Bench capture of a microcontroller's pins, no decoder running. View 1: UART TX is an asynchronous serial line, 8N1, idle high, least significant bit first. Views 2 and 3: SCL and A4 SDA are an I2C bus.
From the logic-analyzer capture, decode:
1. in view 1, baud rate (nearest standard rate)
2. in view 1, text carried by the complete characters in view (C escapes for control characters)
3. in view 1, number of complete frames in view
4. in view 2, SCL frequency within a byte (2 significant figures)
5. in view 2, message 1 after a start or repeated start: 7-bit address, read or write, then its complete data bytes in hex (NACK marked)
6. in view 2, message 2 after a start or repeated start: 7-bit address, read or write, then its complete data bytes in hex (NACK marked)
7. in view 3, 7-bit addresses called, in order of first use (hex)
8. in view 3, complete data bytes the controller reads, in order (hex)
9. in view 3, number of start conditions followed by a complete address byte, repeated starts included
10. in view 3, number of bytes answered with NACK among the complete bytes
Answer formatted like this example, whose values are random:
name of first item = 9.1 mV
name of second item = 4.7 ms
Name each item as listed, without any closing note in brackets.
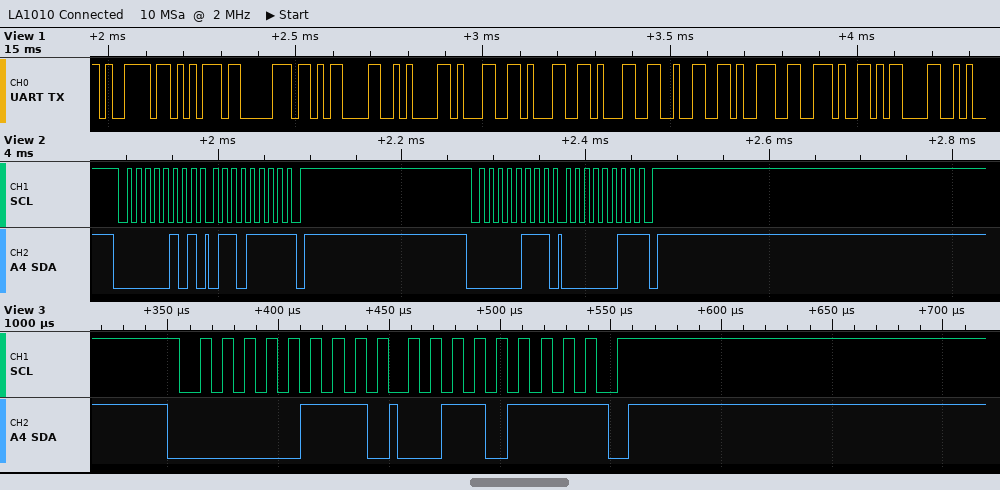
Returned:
in view 1, baud rate = 57600 baud
in view 1, text carried by the complete characters in view = "yup\r\n11129.\r"
in view 1, number of complete frames in view = 12
in view 2, SCL frequency within a byte = 100 kHz
in view 2, message 1 after a start or repeated start: 7-bit address, read or write, then its complete data bytes in hex = 0x02 read: 6F NACK
in view 2, message 2 after a start or repeated start: 7-bit address, read or write, then its complete data bytes in hex = 0x03 read: 03 NACK
in view 3, 7-bit addresses called, in order of first use = 0x03
in view 3, complete data bytes the controller reads, in order = 37
in view 3, number of start conditions followed by a complete address byte, repeated starts included = 1
in view 3, number of bytes answered with NACK among the complete bytes = 1
